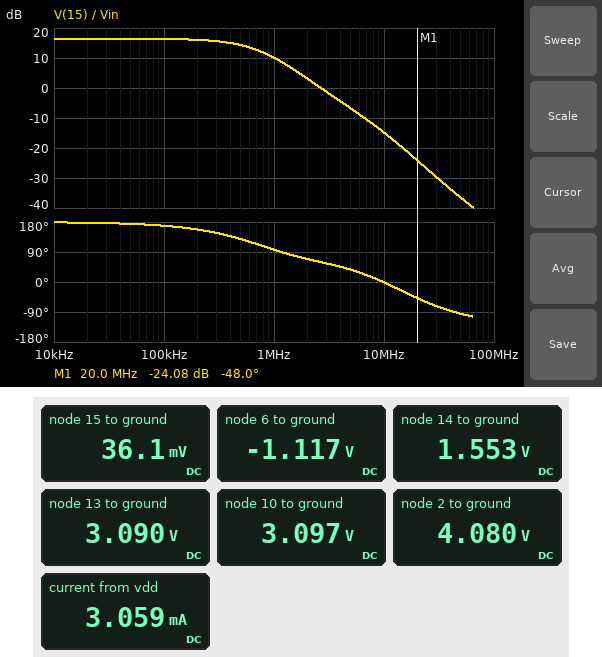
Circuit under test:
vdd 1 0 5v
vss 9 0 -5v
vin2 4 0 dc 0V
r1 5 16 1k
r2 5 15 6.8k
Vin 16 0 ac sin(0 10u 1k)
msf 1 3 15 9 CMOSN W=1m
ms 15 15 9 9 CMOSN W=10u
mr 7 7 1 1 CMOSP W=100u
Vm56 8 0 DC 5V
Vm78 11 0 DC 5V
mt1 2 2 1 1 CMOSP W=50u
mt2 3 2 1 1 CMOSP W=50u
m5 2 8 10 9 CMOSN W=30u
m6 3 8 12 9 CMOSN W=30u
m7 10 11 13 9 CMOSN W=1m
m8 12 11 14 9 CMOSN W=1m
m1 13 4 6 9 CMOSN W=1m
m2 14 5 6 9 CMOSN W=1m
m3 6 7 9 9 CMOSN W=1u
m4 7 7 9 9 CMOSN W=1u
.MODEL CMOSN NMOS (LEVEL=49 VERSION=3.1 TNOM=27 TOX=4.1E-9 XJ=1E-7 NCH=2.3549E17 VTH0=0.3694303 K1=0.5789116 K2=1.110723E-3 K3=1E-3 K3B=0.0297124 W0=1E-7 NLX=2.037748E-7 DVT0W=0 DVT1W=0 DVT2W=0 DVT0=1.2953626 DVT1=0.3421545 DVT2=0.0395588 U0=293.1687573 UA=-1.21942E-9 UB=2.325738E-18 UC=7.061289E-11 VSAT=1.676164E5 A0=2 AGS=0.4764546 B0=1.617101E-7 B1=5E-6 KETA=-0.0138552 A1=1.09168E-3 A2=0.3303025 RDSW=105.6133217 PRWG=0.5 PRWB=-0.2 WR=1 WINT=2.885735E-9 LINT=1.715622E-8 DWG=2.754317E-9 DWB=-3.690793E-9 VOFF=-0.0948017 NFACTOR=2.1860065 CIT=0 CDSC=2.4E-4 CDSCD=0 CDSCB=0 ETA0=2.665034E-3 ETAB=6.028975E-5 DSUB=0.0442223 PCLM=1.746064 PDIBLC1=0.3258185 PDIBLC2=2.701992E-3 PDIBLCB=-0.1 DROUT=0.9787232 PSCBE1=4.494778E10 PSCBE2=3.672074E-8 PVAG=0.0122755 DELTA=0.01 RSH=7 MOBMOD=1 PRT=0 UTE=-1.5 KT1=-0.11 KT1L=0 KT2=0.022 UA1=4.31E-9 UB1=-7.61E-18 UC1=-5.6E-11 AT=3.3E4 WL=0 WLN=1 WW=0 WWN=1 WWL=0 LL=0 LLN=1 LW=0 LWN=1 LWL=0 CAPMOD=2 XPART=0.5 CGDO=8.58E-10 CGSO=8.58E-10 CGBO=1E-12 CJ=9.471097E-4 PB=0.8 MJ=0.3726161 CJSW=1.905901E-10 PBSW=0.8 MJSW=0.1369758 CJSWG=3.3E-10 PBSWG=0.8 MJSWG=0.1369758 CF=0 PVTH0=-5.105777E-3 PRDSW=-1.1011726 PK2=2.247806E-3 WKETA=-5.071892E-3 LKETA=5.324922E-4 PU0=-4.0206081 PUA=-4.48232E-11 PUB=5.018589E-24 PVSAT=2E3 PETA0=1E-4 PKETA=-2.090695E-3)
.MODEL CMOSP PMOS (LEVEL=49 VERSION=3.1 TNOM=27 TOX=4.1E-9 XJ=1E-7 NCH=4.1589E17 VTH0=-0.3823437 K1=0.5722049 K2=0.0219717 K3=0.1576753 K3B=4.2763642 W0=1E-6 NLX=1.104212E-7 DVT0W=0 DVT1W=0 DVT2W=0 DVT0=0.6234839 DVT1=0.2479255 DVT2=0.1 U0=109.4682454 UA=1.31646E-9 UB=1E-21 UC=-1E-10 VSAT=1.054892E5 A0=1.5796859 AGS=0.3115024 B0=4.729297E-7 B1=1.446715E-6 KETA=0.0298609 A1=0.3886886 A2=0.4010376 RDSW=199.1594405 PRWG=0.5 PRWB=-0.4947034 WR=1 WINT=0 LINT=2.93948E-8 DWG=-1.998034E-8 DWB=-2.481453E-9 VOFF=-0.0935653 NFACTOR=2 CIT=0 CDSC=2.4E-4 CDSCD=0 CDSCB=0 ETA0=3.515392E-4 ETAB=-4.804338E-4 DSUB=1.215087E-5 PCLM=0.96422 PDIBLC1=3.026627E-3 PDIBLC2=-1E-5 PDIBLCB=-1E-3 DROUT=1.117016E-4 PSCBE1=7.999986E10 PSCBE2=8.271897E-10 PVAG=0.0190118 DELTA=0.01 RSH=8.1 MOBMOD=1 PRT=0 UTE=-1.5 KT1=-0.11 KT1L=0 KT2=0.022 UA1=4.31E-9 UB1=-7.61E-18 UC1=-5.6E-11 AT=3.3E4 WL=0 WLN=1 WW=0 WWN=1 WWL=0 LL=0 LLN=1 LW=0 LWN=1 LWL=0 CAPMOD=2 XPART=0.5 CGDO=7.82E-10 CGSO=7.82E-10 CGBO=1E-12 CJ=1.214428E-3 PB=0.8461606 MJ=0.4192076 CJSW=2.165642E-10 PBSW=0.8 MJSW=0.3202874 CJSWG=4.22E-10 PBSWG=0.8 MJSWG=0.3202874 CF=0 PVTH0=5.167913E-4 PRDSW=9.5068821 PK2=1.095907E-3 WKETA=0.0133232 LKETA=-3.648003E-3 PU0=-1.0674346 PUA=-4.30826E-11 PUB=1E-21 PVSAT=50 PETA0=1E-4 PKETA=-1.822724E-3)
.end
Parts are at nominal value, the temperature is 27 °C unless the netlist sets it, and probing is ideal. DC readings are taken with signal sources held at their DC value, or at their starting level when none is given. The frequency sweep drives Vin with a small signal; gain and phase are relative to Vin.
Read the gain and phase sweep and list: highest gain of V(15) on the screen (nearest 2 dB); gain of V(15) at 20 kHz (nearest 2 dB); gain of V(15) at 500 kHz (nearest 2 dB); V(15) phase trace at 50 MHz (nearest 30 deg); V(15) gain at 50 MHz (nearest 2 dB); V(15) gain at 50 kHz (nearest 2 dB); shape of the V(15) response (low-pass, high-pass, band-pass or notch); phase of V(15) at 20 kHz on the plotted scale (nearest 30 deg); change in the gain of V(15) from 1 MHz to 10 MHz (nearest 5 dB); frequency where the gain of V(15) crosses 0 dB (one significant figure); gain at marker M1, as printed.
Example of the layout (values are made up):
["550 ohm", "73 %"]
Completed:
["16 dB", "16 dB", "14 dB", "-90 deg", "-36 dB", "16 dB", "low-pass", "180 deg", "-25 dB", "3 MHz", "-24.08 dB"]
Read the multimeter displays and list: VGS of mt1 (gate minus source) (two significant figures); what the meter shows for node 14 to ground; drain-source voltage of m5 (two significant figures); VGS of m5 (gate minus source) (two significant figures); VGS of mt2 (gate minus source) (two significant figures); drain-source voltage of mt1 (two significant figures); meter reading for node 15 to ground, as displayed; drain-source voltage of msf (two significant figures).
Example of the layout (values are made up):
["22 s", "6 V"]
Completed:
["-920 mV", "1.553 V", "980 mV", "1.9 V", "-920 mV", "-920 mV", "36.1 mV", "5.0 V"]
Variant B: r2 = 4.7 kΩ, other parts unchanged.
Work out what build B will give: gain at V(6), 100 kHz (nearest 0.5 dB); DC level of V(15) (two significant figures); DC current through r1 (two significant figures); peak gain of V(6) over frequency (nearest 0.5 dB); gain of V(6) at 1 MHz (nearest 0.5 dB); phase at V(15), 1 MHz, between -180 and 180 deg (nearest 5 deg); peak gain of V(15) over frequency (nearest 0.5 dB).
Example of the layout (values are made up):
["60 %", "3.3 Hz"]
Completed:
["-25.5 dB", "27 mV", "4.7 µA", "-8.0 dB", "-8.5 dB", "105 deg", "13.5 dB"]
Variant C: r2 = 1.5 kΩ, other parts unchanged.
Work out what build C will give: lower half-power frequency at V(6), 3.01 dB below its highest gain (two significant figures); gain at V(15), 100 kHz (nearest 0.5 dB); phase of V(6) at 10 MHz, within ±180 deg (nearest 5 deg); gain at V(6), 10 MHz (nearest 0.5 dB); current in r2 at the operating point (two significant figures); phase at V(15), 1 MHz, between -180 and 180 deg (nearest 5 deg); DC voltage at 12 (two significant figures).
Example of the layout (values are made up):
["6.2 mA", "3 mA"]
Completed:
["1.2 MHz", "3.5 dB", "-25 deg", "-11.5 dB", "4.7 µA", "135 deg", "1.5 V"]
